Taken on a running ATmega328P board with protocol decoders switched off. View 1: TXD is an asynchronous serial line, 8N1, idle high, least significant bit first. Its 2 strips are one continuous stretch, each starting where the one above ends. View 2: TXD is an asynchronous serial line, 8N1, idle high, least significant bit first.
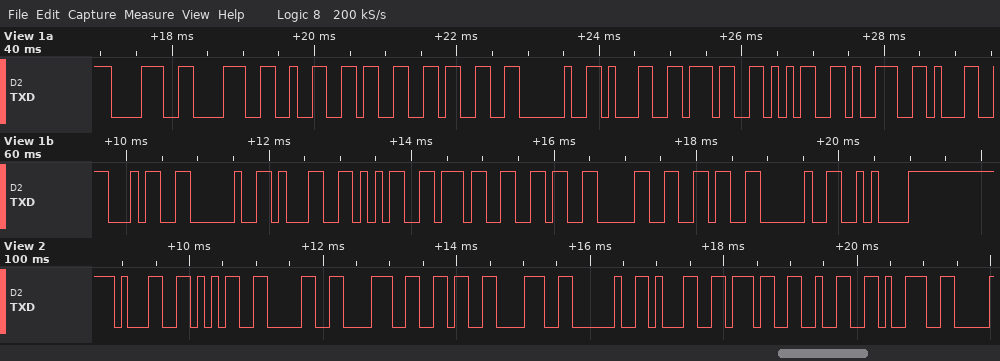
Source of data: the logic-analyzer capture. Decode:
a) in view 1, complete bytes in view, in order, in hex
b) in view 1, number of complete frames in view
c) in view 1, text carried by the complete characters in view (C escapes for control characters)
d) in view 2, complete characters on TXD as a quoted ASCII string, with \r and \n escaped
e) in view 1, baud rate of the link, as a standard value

38 38 32 33 33 20 31 37 35 39 31 34 20 31 35 37 36 30 36 20 0A
21
"88233 175914 157606 \n"
"150868 1729"
9600 baud
